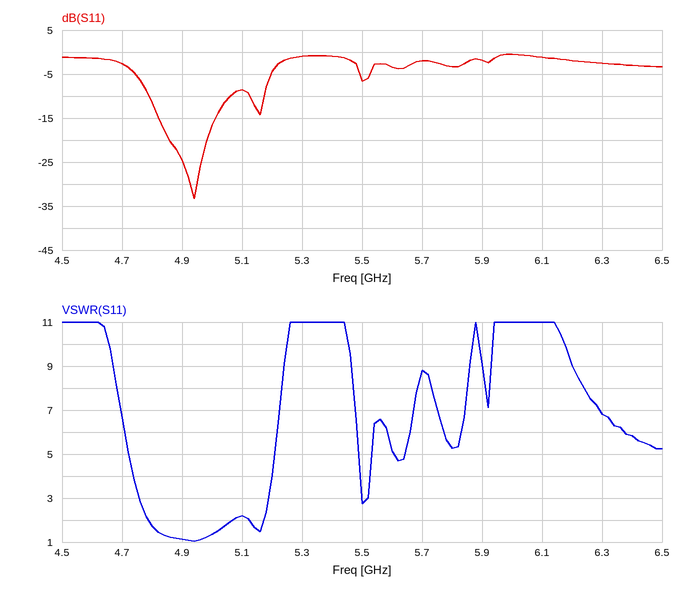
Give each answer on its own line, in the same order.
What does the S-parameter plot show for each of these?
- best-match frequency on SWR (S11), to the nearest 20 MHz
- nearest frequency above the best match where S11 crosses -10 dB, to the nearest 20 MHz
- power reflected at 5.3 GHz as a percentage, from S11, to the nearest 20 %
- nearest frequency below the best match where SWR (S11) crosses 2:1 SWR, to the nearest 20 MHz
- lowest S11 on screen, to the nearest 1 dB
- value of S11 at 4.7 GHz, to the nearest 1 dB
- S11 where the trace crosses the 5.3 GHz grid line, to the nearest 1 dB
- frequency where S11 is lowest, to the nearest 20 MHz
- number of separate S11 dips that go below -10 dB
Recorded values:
4.94 GHz
5.06 GHz
80 %
4.78 GHz
-33 dB
-3 dB
-1 dB
4.94 GHz
2
